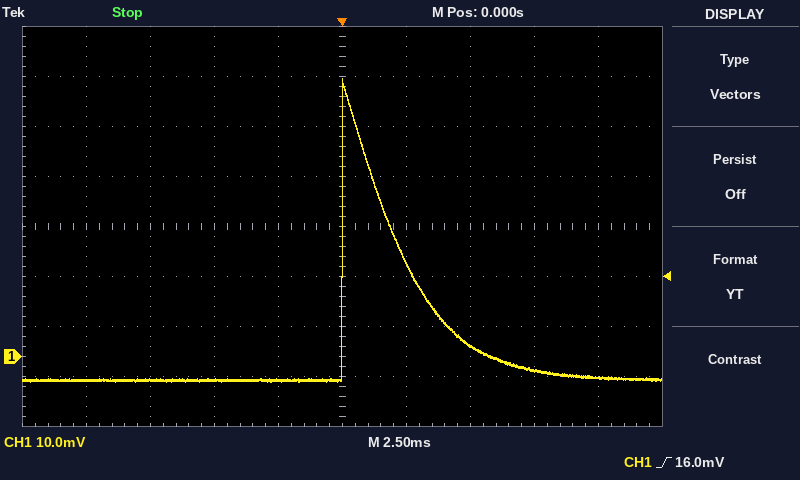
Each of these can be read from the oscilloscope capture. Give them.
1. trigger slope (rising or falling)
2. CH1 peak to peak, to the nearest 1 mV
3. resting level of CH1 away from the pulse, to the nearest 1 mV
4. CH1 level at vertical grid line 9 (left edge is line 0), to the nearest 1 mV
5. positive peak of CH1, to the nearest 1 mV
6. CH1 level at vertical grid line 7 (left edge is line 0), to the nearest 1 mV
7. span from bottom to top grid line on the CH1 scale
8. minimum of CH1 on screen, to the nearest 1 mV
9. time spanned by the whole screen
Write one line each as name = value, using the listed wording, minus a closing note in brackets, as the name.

trigger slope = rising
CH1 peak to peak, to the nearest 1 mV = 61 mV
resting level of CH1 away from the pulse, to the nearest 1 mV = -5 mV
CH1 level at vertical grid line 9 (left edge is line 0), to the nearest 1 mV = -4 mV
positive peak of CH1, to the nearest 1 mV = 56 mV
CH1 level at vertical grid line 7 (left edge is line 0), to the nearest 1 mV = 2 mV
span from bottom to top grid line on the CH1 scale = 80 mV
minimum of CH1 on screen, to the nearest 1 mV = -5 mV
time spanned by the whole screen = 25 ms
